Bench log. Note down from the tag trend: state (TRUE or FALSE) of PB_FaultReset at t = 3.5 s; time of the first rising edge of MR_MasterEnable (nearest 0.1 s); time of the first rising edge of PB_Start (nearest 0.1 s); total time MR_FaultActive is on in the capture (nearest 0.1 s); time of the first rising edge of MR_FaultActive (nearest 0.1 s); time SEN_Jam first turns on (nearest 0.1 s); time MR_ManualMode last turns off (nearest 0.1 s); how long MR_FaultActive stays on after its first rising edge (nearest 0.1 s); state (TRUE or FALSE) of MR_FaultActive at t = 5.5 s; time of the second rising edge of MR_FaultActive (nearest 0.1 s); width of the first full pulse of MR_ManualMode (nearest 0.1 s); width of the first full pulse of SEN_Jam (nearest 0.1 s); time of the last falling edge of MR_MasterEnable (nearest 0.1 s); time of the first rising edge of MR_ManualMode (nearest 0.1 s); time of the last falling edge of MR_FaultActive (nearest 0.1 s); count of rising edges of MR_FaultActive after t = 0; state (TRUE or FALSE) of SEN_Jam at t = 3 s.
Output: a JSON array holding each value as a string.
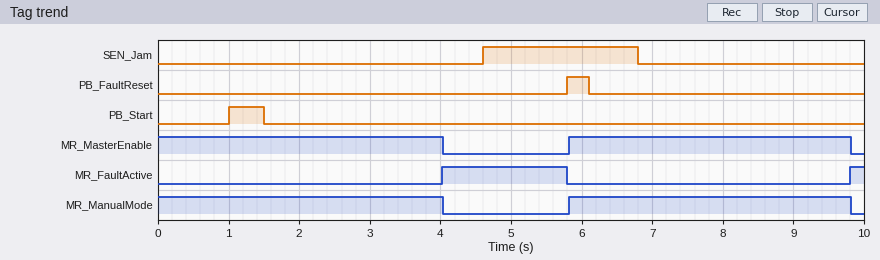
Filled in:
["FALSE", "5.8 s", "1.0 s", "2.0 s", "4.0 s", "4.6 s", "9.8 s", "1.8 s", "TRUE", "9.8 s", "4.0 s", "2.2 s", "9.8 s", "5.8 s", "5.8 s", "2", "FALSE"]
